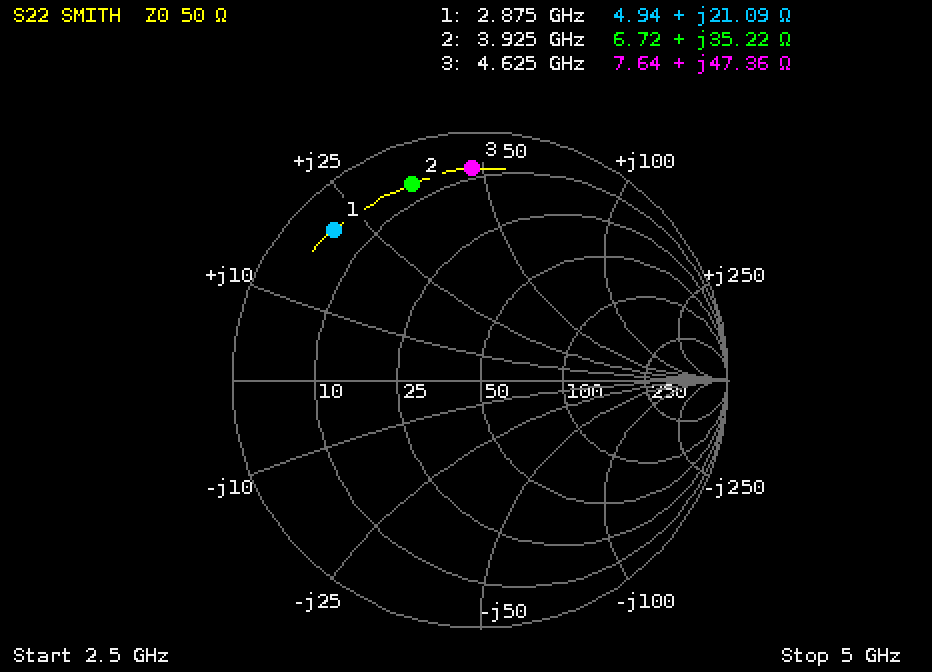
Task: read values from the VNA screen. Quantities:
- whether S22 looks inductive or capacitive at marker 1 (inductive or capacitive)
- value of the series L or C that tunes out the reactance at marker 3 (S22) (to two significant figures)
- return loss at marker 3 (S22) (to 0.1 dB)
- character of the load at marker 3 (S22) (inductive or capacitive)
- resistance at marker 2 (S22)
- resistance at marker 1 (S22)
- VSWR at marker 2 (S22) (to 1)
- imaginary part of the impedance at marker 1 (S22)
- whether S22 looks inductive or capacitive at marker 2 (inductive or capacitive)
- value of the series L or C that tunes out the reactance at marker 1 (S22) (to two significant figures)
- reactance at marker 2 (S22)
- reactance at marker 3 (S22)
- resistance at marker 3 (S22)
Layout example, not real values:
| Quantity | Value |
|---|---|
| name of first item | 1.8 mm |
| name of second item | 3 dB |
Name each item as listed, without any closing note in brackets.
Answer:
| Quantity | Value |
|---|---|
| whether S22 looks inductive or capacitive at marker 1 | inductive |
| value of the series L or C that tunes out the reactance at marker 3 (S22) | 730 fF |
| return loss at marker 3 (S22) | 1.4 dB |
| character of the load at marker 3 (S22) | inductive |
| resistance at marker 2 | 6.72 Ω |
| resistance at marker 1 | 4.94 Ω |
| VSWR at marker 2 (S22) | 11 |
| imaginary part of the impedance at marker 1 | +21.09 Ω |
| whether S22 looks inductive or capacitive at marker 2 | inductive |
| value of the series L or C that tunes out the reactance at marker 1 (S22) | 2.6 pF |
| reactance at marker 2 | +35.22 Ω |
| reactance at marker 3 | +47.36 Ω |
| resistance at marker 3 | 7.64 Ω |
